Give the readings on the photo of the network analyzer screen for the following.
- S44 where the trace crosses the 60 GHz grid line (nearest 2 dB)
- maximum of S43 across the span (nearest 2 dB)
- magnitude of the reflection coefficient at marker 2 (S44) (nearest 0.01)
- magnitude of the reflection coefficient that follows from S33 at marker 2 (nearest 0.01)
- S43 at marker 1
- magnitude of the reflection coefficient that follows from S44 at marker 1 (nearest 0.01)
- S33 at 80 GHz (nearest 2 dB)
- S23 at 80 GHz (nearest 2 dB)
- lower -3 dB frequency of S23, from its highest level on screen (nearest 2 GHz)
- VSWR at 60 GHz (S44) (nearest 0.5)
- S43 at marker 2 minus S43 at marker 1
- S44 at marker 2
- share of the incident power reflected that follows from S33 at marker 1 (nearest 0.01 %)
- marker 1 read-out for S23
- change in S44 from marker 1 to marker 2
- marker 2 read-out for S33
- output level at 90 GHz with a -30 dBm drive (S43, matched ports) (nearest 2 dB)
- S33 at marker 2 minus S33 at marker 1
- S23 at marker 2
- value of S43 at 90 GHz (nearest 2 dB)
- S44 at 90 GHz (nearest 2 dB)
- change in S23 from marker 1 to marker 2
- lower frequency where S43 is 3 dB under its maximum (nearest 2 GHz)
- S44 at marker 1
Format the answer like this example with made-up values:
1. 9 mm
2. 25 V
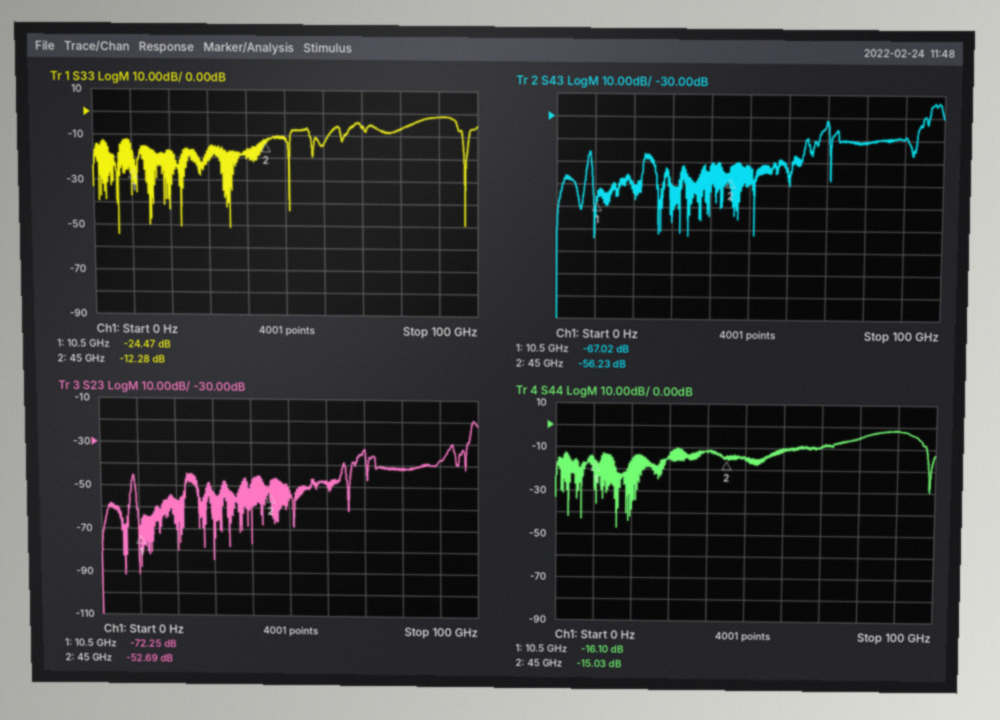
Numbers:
1. -10 dB
2. -24 dB
3. 0.18
4. 0.24
5. -67.02 dB
6. 0.16
7. -6 dB
8. -42 dB
9. 98 GHz
10. 2.0
11. 10.79 dB
12. -15.03 dB
13. 0.36 %
14. -72.25 dB
15. 1.07 dB
16. -12.28 dB
17. -70 dBm
18. 12.19 dB
19. -52.69 dB
20. -40 dB
21. -2 dB
22. 19.56 dB
23. 96 GHz
24. -16.10 dB
